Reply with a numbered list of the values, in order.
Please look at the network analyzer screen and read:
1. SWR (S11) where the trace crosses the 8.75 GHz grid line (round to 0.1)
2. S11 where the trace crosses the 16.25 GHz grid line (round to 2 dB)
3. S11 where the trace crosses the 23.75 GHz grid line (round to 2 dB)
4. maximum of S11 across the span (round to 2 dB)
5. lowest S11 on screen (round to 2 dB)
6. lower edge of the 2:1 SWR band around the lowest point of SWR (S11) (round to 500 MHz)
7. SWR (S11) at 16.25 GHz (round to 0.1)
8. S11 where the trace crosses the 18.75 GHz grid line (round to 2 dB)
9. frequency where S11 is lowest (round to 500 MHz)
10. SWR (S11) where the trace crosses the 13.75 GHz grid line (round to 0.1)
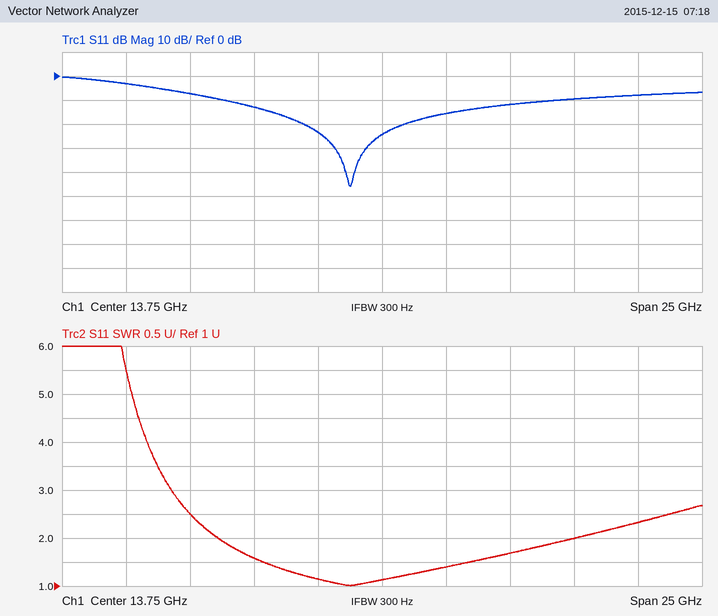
1. 1.6
2. -16 dB
3. -8 dB
4. 0 dB
5. -46 dB
6. 7.5 GHz
7. 1.4
8. -12 dB
9. 12.5 GHz
10. 1.1
